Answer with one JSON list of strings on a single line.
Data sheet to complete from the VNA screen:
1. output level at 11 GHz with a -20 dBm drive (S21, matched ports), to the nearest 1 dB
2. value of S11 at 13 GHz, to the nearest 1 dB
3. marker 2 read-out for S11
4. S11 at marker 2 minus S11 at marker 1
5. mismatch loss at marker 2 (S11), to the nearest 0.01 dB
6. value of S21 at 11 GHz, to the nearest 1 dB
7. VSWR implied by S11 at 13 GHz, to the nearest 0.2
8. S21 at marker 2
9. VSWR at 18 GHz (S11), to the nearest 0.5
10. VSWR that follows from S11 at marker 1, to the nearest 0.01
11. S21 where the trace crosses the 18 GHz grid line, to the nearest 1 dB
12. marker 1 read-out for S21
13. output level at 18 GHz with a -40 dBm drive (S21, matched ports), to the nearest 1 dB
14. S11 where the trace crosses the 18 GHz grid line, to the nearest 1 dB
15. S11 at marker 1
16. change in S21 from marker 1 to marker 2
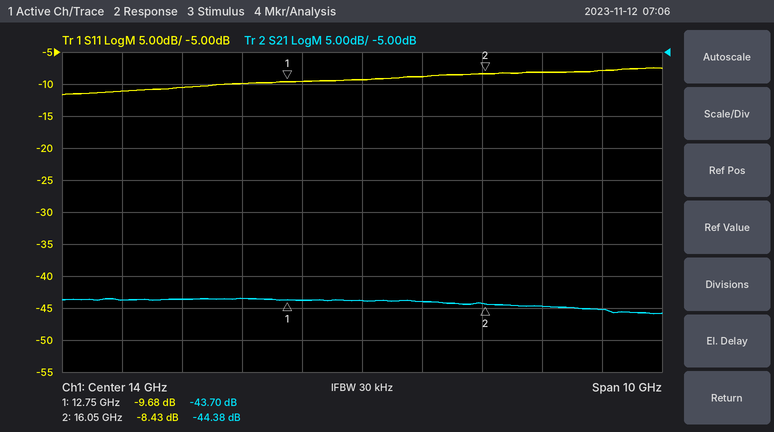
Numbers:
["-64 dBm", "-10 dB", "-8.43 dB", "1.25 dB", "0.67 dB", "-44 dB", "2.0", "-44.38 dB", "2.5", "1.98", "-45 dB", "-43.70 dB", "-85 dBm", "-8 dB", "-9.68 dB", "-0.68 dB"]
